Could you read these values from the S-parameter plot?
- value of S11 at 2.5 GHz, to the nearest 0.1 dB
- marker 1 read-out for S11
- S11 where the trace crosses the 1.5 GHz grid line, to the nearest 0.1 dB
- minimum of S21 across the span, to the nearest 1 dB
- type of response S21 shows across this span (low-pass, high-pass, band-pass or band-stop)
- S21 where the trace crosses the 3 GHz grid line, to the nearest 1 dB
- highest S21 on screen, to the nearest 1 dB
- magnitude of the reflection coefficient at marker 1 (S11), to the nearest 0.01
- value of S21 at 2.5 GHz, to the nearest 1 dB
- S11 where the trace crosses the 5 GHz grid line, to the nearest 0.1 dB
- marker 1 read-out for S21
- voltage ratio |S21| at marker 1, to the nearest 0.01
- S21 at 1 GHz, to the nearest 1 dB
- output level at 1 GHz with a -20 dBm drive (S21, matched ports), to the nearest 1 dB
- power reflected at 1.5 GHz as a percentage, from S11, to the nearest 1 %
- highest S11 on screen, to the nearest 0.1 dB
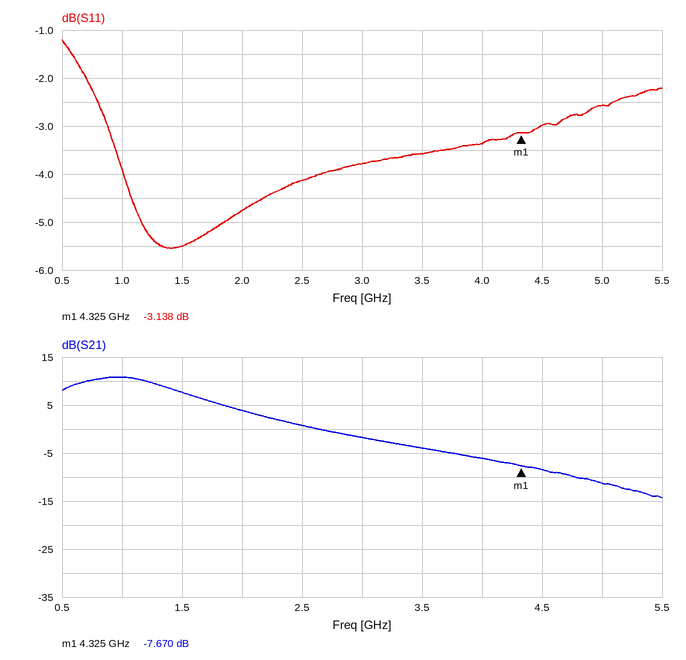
-4.1 dB
-3.138 dB
-5.5 dB
-14 dB
low-pass
-2 dB
11 dB
0.70
1 dB
-2.6 dB
-7.670 dB
0.41
11 dB
-9 dBm
28 %
-1.2 dB
